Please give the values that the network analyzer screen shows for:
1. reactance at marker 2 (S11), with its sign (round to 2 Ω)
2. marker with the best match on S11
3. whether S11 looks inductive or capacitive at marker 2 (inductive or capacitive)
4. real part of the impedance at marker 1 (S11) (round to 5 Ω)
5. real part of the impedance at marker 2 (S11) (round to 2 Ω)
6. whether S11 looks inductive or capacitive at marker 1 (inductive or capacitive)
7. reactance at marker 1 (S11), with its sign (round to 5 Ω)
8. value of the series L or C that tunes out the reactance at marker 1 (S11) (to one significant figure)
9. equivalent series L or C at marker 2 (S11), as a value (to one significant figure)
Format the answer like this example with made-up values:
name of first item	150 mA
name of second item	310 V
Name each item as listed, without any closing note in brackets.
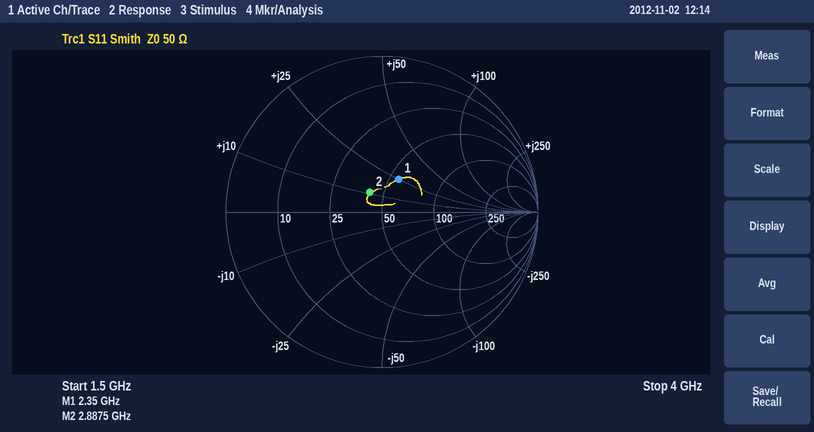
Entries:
reactance at marker 2 (S11), with its sign	+10 Ω
marker with the best match on S11	marker 2
whether S11 looks inductive or capacitive at marker 2	inductive
real part of the impedance at marker 1 (S11)	55 Ω
real part of the impedance at marker 2 (S11)	42 Ω
whether S11 looks inductive or capacitive at marker 1	inductive
reactance at marker 1 (S11), with its sign	+25 Ω
value of the series L or C that tunes out the reactance at marker 1 (S11)	3 pF
equivalent series L or C at marker 2 (S11), as a value	600 pH
